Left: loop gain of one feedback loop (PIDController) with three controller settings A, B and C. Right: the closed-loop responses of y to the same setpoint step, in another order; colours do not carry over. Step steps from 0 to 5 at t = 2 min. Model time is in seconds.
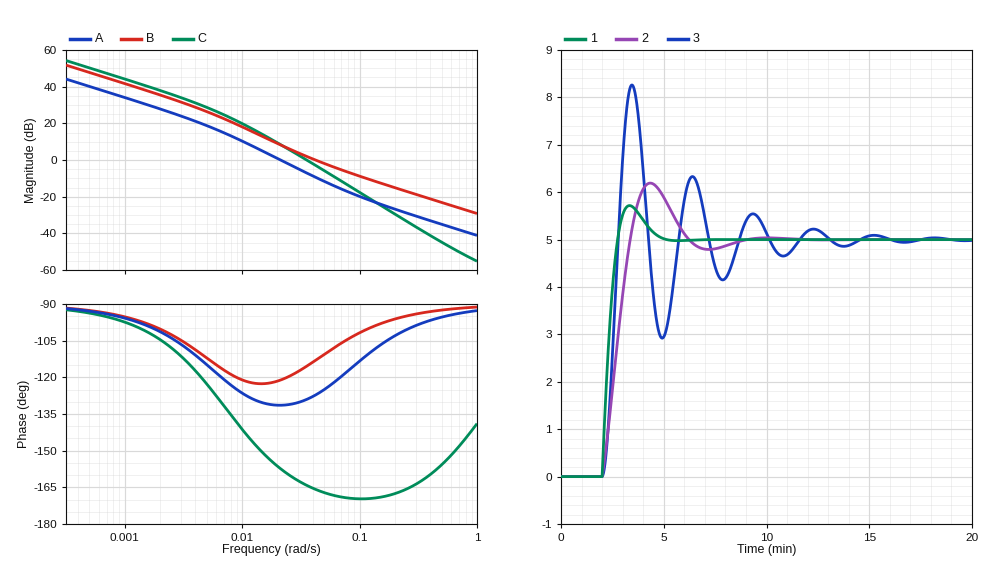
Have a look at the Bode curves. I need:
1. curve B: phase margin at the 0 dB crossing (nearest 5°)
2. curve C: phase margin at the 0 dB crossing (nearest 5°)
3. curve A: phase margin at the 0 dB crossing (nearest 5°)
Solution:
65°
15°
50°
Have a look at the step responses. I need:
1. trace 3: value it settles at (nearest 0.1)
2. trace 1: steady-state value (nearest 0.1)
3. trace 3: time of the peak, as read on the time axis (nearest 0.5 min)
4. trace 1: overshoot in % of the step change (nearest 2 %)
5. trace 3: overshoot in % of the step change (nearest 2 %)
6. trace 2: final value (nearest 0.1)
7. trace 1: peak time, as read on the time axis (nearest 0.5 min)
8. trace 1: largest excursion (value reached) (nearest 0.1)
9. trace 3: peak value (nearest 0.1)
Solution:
5.0
5.0
3.5 min
14 %
66 %
5.0
3.5 min
5.7
8.3
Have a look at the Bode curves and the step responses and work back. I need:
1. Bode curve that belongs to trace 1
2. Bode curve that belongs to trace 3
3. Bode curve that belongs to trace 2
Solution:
B
C
A
